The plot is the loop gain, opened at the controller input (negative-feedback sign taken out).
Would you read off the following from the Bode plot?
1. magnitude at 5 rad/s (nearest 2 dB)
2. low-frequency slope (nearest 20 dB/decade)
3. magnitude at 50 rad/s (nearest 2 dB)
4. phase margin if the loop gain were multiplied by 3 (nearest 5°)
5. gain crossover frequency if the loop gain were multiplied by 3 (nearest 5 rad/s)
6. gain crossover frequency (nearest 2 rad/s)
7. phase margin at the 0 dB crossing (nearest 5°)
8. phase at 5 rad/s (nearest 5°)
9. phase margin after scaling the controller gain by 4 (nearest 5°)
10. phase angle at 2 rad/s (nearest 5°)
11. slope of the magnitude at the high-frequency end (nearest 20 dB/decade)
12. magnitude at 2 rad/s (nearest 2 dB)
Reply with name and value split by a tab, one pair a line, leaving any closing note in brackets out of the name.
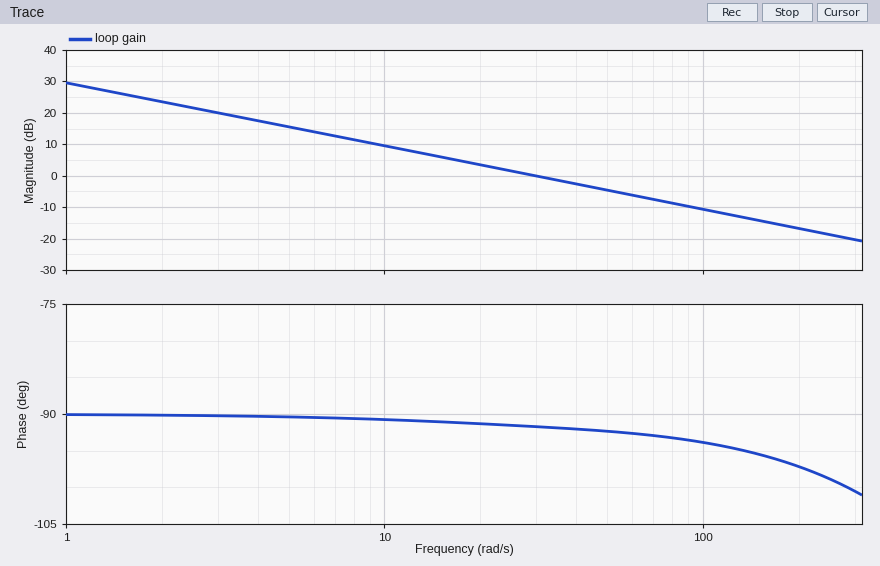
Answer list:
magnitude at 5 rad/s	16 dB
low-frequency slope	-20 dB/decade
magnitude at 50 rad/s	-4 dB
phase margin if the loop gain were multiplied by 3	85°
gain crossover frequency if the loop gain were multiplied by 3	90 rad/s
gain crossover frequency	30 rad/s
phase margin at the 0 dB crossing	90°
phase at 5 rad/s	-90°
phase margin after scaling the controller gain by 4	85°
phase angle at 2 rad/s	-90°
slope of the magnitude at the high-frequency end	-20 dB/decade
magnitude at 2 rad/s	24 dB
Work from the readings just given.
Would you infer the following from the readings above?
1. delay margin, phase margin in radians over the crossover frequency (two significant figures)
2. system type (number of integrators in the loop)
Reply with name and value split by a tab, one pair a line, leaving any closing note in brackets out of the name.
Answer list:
delay margin, phase margin in radians over the crossover frequency	0.052 s
system type	1
